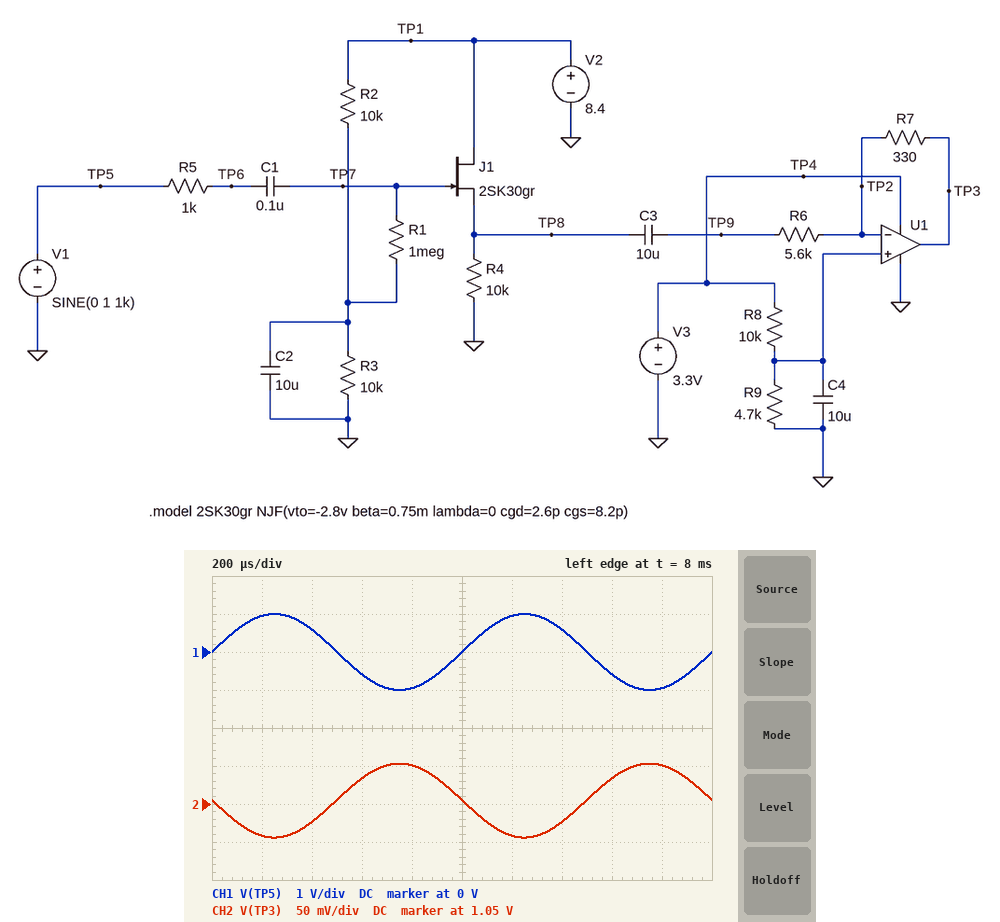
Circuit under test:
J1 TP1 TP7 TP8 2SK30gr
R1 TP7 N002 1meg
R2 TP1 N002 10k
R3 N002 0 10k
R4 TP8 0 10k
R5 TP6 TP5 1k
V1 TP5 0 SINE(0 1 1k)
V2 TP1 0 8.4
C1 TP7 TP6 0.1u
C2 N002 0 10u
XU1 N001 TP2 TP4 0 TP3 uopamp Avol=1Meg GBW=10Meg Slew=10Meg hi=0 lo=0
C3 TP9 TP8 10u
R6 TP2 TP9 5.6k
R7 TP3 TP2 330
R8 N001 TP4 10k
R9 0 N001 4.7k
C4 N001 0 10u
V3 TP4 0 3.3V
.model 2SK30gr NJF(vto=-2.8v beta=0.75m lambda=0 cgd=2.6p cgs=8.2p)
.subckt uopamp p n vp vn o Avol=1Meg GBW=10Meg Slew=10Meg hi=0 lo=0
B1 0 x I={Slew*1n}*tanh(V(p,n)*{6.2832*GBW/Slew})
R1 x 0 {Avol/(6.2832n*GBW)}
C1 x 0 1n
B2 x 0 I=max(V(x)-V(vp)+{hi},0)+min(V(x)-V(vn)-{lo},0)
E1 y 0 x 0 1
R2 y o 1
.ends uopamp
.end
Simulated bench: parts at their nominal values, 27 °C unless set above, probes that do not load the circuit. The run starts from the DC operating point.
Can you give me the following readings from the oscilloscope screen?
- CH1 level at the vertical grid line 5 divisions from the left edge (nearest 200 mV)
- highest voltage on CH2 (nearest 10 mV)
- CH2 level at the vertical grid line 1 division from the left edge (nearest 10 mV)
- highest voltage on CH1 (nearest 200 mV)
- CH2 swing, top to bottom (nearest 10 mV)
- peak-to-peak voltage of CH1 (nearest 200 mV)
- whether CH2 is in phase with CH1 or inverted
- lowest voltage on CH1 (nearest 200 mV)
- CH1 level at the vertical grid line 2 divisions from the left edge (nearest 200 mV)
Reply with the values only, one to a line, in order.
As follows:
0 V
1.10 V
1.01 V
1.0 V
100 mV
2.0 V
inverted
-1.0 V
600 mV
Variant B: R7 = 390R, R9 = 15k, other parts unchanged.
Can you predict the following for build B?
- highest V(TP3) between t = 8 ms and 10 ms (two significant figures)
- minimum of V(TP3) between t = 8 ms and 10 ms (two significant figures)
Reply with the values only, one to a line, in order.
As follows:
2.0 V
1.9 V
